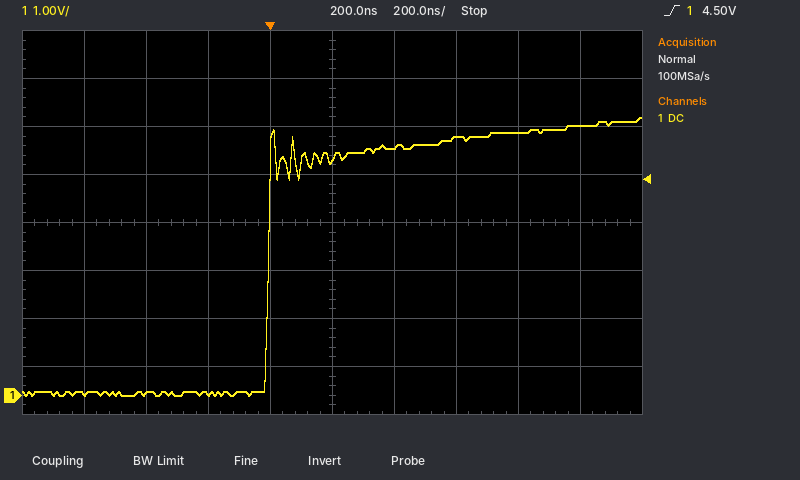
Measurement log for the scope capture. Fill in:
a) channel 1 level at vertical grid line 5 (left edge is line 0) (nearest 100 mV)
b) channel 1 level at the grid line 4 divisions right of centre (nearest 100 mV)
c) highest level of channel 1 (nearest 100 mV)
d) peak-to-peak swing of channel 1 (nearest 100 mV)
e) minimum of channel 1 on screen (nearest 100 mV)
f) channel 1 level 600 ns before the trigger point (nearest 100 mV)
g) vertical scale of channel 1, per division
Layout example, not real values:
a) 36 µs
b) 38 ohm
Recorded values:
a) 4.9 V
b) 5.6 V
c) 5.8 V
d) 5.8 V
e) 0.0 V
f) 0.0 V
g) 1 V
